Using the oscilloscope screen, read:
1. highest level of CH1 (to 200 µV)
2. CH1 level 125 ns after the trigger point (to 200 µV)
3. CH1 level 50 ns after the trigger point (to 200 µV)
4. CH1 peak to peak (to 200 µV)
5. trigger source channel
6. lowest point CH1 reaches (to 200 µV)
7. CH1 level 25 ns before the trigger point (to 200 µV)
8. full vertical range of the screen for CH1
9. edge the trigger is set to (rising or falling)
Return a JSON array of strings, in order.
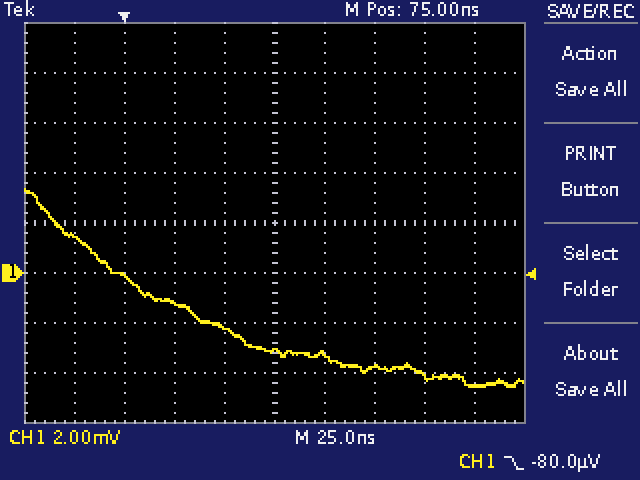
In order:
["3.4 mV", "-3.8 mV", "-2.2 mV", "8.0 mV", "CH1", "-4.6 mV", "1.4 mV", "16 mV", "falling"]
